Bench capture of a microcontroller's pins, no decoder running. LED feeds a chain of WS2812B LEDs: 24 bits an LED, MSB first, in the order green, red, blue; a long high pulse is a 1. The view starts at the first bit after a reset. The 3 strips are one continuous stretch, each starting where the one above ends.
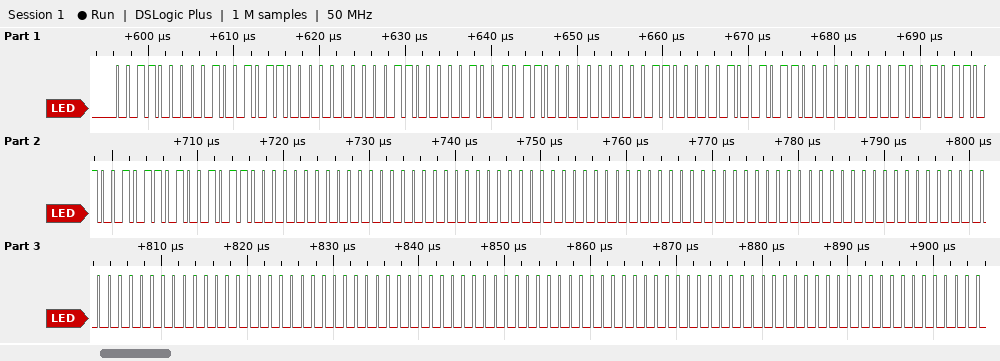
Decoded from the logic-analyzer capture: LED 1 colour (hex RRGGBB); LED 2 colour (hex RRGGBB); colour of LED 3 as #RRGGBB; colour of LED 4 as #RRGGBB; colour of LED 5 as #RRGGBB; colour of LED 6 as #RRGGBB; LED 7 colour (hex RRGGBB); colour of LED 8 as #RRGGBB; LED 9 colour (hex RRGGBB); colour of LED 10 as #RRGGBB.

#4B3000
#4B3000
#4B3000
#4B4B4B
#000000
#000000
#000000
#000000
#000000
#000000
